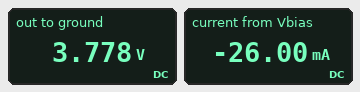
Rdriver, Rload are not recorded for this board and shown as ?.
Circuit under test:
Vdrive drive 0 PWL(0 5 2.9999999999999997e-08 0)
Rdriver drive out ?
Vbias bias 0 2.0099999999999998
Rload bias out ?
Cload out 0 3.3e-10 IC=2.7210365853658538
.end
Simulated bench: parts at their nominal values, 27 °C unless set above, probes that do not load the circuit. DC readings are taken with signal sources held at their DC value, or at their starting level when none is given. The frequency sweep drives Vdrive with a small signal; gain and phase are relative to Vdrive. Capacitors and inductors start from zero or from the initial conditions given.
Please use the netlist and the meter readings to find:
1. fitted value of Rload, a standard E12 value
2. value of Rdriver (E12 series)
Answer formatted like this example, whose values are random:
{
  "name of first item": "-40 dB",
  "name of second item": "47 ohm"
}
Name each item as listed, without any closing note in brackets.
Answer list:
{
  "fitted value of Rload, a standard E12 value": "68 Ω",
  "value of Rdriver": "47 Ω"
}
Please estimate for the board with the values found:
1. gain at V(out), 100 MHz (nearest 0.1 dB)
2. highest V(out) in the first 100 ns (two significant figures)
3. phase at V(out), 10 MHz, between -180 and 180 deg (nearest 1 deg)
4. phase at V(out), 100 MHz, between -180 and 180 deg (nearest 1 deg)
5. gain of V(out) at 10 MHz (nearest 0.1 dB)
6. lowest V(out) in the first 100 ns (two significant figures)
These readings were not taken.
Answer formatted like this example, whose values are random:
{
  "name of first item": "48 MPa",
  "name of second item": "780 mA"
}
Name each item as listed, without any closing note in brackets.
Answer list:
{
  "gain at V(out), 100 MHz": "-19.9 dB",
  "highest V(out) in the first 100 ns": "3.1 V",
  "phase at V(out), 10 MHz, between -180 and 180 deg": "-30 deg",
  "phase at V(out), 100 MHz, between -180 and 180 deg": "-80 deg",
  "gain of V(out) at 10 MHz": "-5.8 dB",
  "lowest V(out) in the first 100 ns": "820 mV"
}
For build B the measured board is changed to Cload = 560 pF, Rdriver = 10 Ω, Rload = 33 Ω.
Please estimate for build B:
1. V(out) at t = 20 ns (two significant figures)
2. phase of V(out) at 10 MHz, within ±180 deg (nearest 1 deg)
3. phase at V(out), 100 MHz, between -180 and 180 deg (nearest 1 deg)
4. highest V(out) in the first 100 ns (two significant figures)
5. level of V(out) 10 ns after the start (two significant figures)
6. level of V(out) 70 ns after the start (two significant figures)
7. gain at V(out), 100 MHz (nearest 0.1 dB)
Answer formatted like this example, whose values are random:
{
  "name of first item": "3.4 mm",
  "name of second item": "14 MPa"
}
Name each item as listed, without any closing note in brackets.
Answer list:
{
  "V(out) at t = 20 ns": "2.3 V",
  "phase of V(out) at 10 MHz, within ±180 deg": "-15 deg",
  "phase at V(out), 100 MHz, between -180 and 180 deg": "-70 deg",
  "highest V(out) in the first 100 ns": "3.6 V",
  "level of V(out) 10 ns after the start": "3.4 V",
  "level of V(out) 70 ns after the start": "470 mV",
  "gain at V(out), 100 MHz": "-11.5 dB"
}
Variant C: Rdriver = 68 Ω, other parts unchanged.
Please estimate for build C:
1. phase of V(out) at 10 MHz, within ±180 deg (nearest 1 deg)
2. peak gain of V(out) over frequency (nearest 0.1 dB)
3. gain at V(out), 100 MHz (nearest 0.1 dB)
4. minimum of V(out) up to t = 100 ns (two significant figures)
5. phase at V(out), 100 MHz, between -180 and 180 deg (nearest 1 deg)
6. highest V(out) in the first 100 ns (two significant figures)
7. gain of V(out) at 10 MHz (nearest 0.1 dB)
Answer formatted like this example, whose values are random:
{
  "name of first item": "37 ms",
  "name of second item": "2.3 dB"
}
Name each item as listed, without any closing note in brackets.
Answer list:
{
  "phase of V(out) at 10 MHz, within ±180 deg": "-35 deg",
  "peak gain of V(out) over frequency": "-6.0 dB",
  "gain at V(out), 100 MHz": "-23.1 dB",
  "minimum of V(out) up to t = 100 ns": "1.0 V",
  "phase at V(out), 100 MHz, between -180 and 180 deg": "-82 deg",
  "highest V(out) in the first 100 ns": "2.9 V",
  "gain of V(out) at 10 MHz": "-7.8 dB"
}
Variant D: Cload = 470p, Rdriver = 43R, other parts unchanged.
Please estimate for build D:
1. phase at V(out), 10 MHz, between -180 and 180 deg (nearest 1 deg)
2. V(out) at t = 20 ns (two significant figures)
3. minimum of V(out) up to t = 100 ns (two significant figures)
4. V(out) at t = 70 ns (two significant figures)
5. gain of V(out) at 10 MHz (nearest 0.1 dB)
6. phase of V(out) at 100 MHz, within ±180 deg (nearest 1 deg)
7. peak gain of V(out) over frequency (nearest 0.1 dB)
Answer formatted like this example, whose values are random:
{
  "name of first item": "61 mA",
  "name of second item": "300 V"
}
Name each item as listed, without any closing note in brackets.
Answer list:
{
  "phase at V(out), 10 MHz, between -180 and 180 deg": "-38 deg",
  "V(out) at t = 20 ns": "2.6 V",
  "minimum of V(out) up to t = 100 ns": "780 mV",
  "V(out) at t = 70 ns": "820 mV",
  "gain of V(out) at 10 MHz": "-6.3 dB",
  "phase of V(out) at 100 MHz, within ±180 deg": "-83 deg",
  "peak gain of V(out) over frequency": "-4.3 dB"
}
